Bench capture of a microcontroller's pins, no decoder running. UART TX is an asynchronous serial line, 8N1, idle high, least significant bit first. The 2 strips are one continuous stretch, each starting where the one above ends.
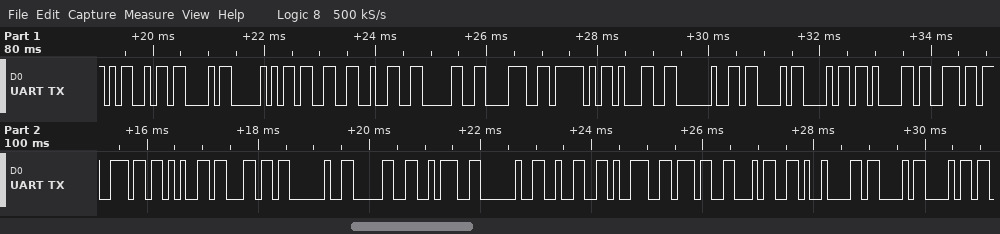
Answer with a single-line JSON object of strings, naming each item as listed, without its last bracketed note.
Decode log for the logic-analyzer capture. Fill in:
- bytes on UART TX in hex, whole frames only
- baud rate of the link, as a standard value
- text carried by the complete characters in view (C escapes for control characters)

{"bytes on UART TX in hex, whole frames only": "4D 43 50 33 32 30 38 5F 31 20 43 68 61 6E 6E 65 6C 20 30 3A 20 32 39 37 34 09 43 68", "baud rate of the link, as a standard value": "9600 baud", "text carried by the complete characters in view": "\"MCP3208_1 Channel 0: 2974\\tCh\""}
